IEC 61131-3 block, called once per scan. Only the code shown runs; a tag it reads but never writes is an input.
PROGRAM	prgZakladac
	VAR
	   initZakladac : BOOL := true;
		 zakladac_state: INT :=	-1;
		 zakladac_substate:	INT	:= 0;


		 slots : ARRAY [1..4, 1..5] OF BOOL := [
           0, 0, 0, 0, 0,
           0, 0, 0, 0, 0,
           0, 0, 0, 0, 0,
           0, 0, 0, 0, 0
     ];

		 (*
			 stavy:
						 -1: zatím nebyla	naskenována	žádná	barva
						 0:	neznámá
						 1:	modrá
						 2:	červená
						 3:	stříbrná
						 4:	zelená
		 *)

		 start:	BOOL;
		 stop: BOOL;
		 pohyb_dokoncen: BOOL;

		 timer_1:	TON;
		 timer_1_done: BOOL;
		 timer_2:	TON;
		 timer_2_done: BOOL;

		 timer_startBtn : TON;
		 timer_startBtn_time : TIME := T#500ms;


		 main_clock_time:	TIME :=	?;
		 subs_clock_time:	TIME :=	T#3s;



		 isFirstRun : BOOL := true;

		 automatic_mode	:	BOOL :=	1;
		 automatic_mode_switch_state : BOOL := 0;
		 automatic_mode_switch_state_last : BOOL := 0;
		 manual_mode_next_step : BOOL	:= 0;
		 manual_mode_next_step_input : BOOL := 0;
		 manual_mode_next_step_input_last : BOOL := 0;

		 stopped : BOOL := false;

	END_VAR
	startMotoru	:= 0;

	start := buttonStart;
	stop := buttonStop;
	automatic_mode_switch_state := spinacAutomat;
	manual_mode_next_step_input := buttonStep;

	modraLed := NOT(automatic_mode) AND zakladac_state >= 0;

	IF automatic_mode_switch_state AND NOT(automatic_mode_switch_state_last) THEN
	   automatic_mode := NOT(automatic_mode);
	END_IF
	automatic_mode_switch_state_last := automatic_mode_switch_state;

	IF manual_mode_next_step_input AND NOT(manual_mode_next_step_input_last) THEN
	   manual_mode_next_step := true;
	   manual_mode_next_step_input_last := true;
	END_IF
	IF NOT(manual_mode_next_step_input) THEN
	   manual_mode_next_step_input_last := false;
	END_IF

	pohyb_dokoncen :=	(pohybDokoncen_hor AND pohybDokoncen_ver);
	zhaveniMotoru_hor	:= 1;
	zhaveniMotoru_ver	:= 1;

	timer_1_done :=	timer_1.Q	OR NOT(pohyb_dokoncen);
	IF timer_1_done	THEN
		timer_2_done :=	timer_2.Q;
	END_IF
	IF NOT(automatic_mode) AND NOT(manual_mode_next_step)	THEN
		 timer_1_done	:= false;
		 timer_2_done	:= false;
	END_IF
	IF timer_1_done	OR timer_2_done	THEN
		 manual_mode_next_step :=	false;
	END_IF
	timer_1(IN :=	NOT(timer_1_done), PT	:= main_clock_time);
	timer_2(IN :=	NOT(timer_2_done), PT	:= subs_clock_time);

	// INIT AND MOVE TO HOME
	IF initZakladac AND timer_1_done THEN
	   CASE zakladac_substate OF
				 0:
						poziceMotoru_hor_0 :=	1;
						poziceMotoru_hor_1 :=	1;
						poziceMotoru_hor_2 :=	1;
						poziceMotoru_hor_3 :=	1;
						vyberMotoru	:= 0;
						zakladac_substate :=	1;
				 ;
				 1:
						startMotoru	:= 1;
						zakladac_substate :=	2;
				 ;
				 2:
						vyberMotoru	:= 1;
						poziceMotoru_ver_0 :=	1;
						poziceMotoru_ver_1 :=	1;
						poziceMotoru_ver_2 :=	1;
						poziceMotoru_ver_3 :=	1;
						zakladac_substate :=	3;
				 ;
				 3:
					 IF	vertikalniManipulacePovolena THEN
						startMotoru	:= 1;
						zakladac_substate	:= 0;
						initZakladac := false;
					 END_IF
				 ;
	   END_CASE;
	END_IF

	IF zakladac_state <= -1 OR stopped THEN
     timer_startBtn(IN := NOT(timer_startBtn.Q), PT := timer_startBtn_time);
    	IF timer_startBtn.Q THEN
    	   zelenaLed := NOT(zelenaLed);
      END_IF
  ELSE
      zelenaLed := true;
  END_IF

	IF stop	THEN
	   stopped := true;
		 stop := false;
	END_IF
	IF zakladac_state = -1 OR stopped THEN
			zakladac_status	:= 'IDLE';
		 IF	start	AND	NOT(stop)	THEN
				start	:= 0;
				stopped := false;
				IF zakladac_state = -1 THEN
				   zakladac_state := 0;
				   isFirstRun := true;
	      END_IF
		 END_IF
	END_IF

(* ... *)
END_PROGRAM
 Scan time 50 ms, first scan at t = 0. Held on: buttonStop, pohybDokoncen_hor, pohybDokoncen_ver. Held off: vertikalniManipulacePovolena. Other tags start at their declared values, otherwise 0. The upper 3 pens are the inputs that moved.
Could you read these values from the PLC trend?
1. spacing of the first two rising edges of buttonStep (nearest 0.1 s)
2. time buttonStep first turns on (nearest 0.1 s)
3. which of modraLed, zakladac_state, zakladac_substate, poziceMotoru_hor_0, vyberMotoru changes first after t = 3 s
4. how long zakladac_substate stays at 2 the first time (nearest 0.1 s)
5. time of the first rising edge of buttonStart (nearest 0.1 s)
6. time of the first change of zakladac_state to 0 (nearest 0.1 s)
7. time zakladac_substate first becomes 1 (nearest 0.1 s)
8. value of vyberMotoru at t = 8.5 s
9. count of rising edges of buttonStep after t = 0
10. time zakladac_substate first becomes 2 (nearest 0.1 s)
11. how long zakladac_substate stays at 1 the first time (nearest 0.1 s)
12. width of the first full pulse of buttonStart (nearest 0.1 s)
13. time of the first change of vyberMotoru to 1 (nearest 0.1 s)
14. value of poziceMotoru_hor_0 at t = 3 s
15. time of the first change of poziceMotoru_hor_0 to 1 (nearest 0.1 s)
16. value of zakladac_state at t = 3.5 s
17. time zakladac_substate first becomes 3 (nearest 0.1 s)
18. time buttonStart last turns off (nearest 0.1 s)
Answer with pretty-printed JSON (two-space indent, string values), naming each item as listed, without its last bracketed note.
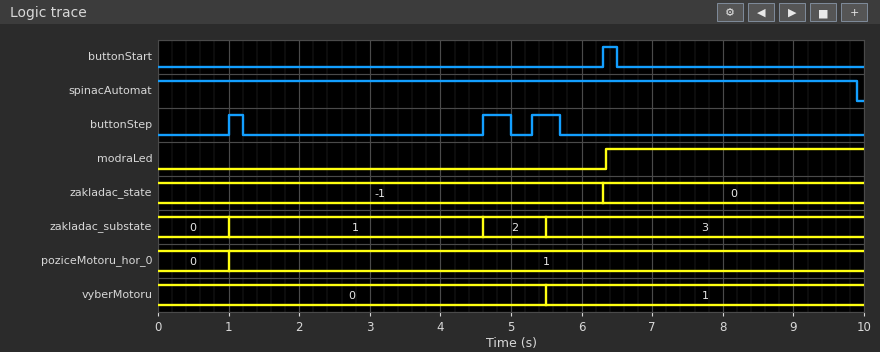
{
  "spacing of the first two rising edges of buttonStep": "3.6 s",
  "time buttonStep first turns on": "1.0 s",
  "which of modraLed, zakladac_state, zakladac_substate, poziceMotoru_hor_0, vyberMotoru changes first after t = 3 s": "zakladac_substate",
  "how long zakladac_substate stays at 2 the first time": "0.9 s",
  "time of the first rising edge of buttonStart": "6.3 s",
  "time of the first change of zakladac_state to 0": "6.3 s",
  "time zakladac_substate first becomes 1": "1.0 s",
  "value of vyberMotoru at t = 8.5 s": "1",
  "count of rising edges of buttonStep after t = 0": "3",
  "time zakladac_substate first becomes 2": "4.6 s",
  "how long zakladac_substate stays at 1 the first time": "3.6 s",
  "width of the first full pulse of buttonStart": "0.2 s",
  "time of the first change of vyberMotoru to 1": "5.5 s",
  "value of poziceMotoru_hor_0 at t = 3 s": "1",
  "time of the first change of poziceMotoru_hor_0 to 1": "1.0 s",
  "value of zakladac_state at t = 3.5 s": "-1",
  "time zakladac_substate first becomes 3": "5.5 s",
  "time buttonStart last turns off": "6.5 s"
}
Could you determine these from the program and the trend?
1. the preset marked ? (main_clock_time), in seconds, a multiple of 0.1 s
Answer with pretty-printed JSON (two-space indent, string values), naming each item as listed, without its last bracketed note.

{
  "the preset marked ? (main_clock_time), in seconds, a multiple of 0.1 s": "0.8 s"
}
